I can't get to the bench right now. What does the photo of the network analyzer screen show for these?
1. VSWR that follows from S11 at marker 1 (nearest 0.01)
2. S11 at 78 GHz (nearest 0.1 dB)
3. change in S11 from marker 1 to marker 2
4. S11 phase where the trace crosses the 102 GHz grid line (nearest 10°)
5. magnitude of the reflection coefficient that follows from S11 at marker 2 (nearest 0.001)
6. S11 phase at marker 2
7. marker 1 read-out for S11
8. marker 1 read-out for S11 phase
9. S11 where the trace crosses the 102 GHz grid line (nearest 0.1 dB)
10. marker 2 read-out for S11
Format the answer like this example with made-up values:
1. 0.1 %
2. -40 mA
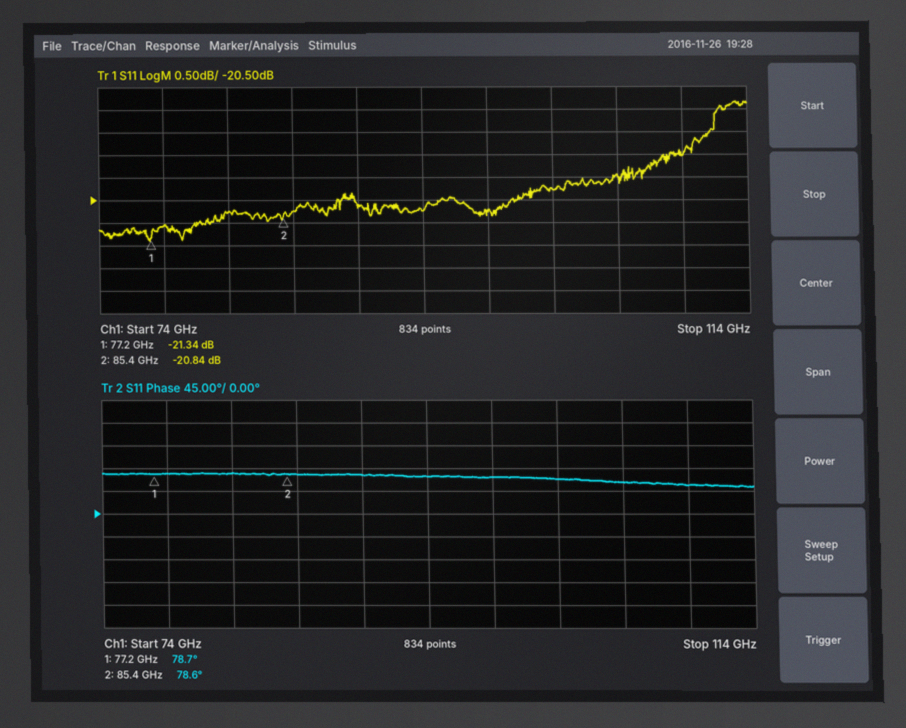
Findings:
1. 1.19
2. -21.1 dB
3. 0.50 dB
4. 70°
5. 0.091
6. 78.6°
7. -21.34 dB
8. 78.7°
9. -20.3 dB
10. -20.84 dB
